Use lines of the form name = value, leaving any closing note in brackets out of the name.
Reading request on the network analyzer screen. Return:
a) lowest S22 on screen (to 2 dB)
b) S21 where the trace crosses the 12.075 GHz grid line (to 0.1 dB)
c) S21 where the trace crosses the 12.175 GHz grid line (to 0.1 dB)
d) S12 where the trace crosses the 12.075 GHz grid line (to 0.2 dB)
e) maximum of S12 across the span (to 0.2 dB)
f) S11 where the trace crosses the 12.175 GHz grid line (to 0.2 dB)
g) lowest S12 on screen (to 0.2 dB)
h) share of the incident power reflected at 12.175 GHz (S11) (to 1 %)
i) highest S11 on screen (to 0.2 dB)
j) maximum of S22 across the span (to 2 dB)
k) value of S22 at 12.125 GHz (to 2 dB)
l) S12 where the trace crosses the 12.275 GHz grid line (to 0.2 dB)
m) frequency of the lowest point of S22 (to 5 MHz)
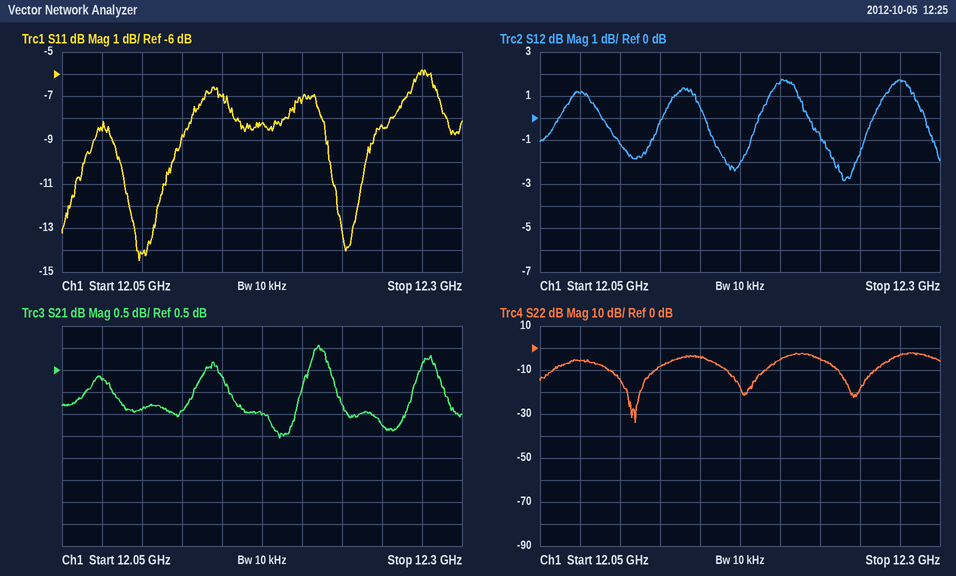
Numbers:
lowest S22 on screen = -34 dB
S21 where the trace crosses the 12.075 GHz grid line = 0.3 dB
S21 where the trace crosses the 12.175 GHz grid line = -0.5 dB
S12 where the trace crosses the 12.075 GHz grid line = 1.2 dB
maximum of S12 across the span = 1.8 dB
S11 where the trace crosses the 12.175 GHz grid line = -8.2 dB
lowest S12 on screen = -2.8 dB
share of the incident power reflected at 12.175 GHz (S11) = 15 %
highest S11 on screen = -5.8 dB
maximum of S22 across the span = -2 dB
value of S22 at 12.125 GHz = -8 dB
S12 where the trace crosses the 12.275 GHz grid line = 1.8 dB
frequency of the lowest point of S22 = 12.110 GHz
